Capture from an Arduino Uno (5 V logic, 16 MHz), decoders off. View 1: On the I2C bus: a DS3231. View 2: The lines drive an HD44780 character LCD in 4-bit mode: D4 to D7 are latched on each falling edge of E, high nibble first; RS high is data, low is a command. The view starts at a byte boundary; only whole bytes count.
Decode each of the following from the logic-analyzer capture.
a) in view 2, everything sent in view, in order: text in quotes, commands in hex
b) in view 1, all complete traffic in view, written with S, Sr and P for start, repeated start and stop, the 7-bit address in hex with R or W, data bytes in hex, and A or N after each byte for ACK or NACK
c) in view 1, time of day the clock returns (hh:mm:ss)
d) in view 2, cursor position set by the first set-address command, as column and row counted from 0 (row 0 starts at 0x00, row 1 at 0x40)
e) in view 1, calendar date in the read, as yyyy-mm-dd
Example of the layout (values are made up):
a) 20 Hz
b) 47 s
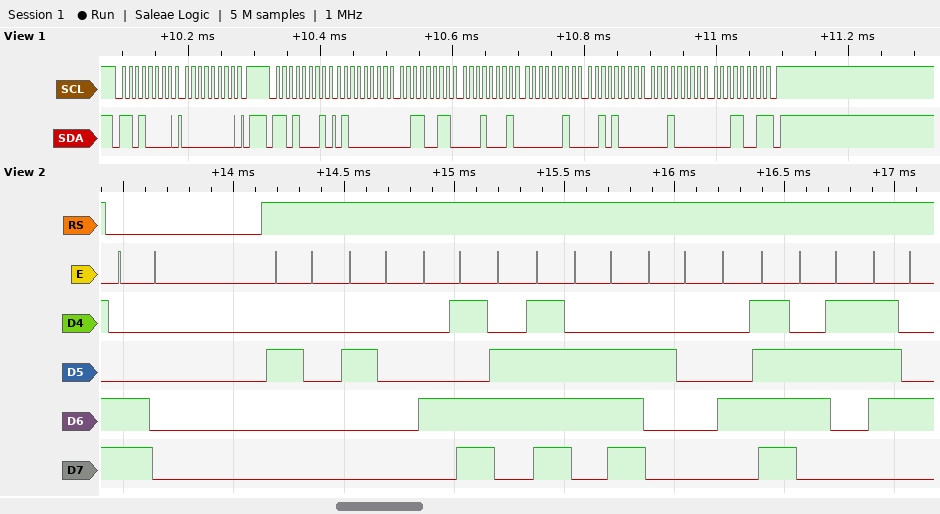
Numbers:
a) 0xC0 "  Mon Oct"
b) S 68W A 00 A P S 68R A 40 A 33 A 11 A 02 A 28 A 10 A 19 N P
c) 11:33:40
d) column 0, row 1
e) 2019-10-28
